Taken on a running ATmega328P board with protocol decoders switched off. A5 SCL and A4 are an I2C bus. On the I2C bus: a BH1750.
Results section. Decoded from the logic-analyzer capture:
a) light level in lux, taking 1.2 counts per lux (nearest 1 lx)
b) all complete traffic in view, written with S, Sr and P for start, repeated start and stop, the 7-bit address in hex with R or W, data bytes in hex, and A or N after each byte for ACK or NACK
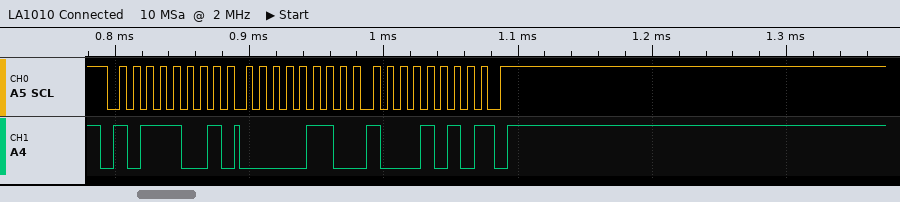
1395 lx
S 5CR A 06 A 8A N P
